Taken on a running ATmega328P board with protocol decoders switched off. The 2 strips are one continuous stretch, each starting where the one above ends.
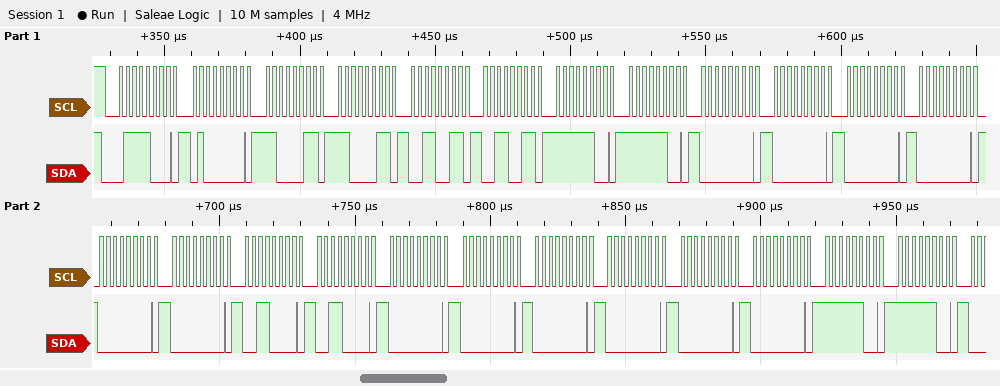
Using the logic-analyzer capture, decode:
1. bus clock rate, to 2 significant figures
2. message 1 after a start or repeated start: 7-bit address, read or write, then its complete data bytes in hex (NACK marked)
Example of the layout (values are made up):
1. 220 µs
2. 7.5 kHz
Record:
1. 400 kHz
2. 0x3C write: 40 C3 C3 33 33 FC FC 00 00 00 00 00 00 30 30 00 00 00 00 00 00 FC FC
